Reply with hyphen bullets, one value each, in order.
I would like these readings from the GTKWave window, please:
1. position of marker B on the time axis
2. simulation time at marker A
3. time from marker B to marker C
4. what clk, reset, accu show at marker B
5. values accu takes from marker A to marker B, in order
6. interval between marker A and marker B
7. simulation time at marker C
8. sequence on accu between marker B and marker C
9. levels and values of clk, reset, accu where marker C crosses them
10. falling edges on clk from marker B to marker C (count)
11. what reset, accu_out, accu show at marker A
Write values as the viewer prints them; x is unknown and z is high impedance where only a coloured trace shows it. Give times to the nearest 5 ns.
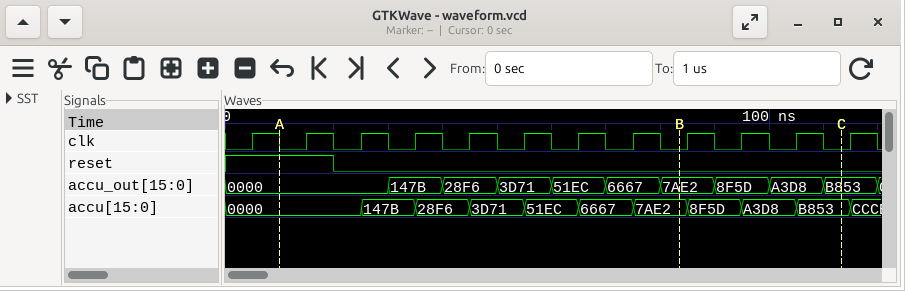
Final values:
- 85 ns
- 10 ns
- 30 ns
- clk=0, reset=0, accu=7AE2
- 0000, 147B, 28F6, 3D71, 51EC, 6667, 7AE2
- 75 ns
- 115 ns
- 7AE2, 8F5D, A3D8, B853
- clk=0, reset=0, accu=B853
- 3
- reset=1, accu_out=0000, accu=0000
